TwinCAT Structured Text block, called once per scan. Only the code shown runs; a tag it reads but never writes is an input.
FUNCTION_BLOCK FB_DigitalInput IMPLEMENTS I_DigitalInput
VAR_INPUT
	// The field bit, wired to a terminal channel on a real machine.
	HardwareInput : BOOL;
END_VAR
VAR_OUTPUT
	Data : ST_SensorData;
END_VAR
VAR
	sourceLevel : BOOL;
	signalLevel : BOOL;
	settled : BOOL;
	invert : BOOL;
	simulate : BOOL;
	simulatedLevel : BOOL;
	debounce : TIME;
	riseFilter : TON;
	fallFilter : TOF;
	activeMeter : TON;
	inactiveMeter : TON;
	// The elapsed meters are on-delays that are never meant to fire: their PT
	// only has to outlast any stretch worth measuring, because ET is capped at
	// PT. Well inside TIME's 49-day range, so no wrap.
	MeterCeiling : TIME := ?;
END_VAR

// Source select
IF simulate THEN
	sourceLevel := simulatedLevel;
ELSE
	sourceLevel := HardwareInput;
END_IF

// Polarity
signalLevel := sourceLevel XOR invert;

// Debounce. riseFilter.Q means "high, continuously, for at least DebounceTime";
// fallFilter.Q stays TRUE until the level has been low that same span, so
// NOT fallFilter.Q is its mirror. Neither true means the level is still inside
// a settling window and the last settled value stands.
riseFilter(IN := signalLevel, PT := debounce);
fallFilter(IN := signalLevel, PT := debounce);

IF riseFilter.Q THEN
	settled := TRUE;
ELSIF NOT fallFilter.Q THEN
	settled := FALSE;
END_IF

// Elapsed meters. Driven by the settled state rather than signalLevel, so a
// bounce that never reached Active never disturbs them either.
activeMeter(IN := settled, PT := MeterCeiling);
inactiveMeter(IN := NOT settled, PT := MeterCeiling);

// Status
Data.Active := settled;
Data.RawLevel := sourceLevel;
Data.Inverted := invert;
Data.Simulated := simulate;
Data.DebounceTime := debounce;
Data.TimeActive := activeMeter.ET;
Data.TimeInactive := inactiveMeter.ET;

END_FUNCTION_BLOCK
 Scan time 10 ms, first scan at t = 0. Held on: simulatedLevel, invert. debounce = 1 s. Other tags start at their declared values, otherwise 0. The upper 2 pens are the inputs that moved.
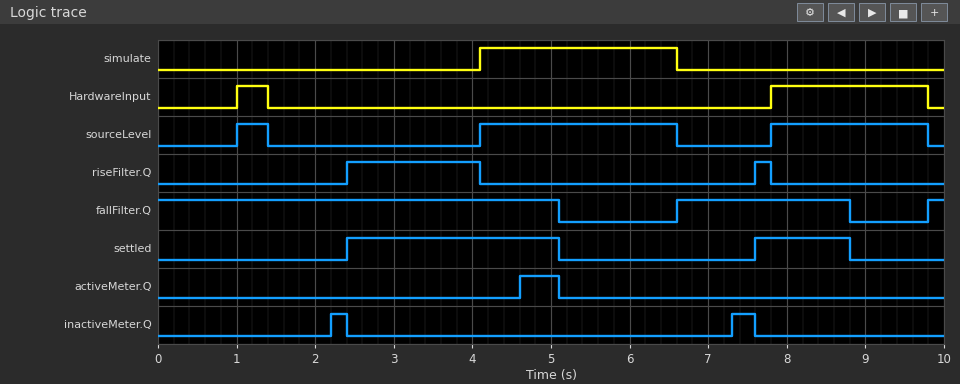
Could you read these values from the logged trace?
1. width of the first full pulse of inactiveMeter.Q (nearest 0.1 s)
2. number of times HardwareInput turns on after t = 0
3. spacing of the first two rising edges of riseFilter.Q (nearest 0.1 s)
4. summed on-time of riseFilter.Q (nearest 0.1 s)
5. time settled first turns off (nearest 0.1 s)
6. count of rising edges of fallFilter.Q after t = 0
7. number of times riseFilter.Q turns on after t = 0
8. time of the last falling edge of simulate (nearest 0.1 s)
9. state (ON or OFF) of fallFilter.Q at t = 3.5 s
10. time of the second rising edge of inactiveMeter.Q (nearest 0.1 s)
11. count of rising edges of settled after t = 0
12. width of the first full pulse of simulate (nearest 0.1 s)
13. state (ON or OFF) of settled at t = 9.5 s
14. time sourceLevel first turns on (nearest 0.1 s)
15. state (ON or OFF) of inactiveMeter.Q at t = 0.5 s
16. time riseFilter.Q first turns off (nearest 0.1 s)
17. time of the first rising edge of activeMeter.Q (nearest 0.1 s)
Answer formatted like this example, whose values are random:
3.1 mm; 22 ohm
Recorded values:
0.2 s; 2; 5.2 s; 1.9 s; 5.1 s; 2; 2; 6.6 s; ON; 7.3 s; 2; 2.5 s; OFF; 1.0 s; OFF; 4.1 s; 4.6 s
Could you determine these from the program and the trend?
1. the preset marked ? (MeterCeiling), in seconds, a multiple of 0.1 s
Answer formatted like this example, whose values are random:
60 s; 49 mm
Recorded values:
2.2 s
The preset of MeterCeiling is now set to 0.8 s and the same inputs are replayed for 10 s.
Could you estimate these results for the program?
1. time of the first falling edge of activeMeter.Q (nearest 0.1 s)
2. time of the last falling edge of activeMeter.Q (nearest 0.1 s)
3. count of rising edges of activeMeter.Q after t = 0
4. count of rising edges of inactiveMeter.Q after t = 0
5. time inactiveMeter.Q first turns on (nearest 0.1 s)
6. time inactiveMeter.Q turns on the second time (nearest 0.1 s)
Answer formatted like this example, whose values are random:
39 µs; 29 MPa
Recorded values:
5.1 s; 8.8 s; 2; 3; 0.8 s; 5.9 s
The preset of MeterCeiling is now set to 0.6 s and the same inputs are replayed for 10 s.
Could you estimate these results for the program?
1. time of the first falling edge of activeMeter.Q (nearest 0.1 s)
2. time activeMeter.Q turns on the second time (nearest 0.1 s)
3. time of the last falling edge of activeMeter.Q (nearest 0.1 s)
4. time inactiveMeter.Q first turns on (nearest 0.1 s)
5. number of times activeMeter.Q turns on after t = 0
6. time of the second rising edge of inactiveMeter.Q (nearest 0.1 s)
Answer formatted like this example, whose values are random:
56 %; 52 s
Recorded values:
5.1 s; 8.2 s; 8.8 s; 0.6 s; 2; 5.7 s
